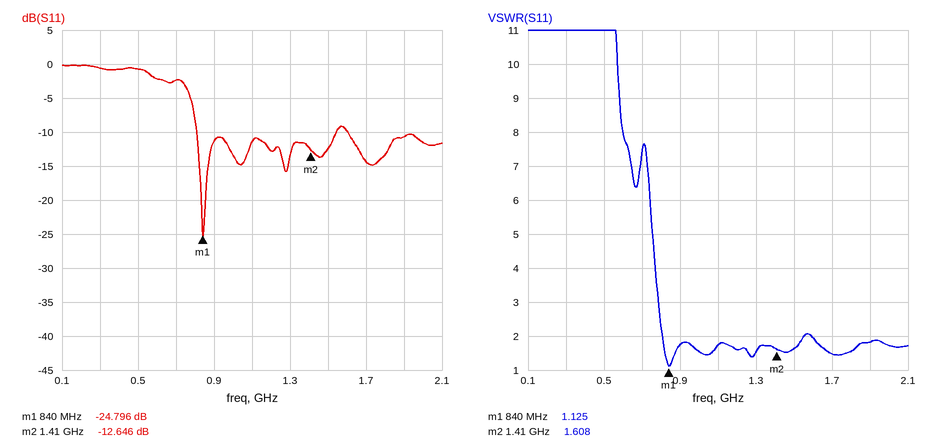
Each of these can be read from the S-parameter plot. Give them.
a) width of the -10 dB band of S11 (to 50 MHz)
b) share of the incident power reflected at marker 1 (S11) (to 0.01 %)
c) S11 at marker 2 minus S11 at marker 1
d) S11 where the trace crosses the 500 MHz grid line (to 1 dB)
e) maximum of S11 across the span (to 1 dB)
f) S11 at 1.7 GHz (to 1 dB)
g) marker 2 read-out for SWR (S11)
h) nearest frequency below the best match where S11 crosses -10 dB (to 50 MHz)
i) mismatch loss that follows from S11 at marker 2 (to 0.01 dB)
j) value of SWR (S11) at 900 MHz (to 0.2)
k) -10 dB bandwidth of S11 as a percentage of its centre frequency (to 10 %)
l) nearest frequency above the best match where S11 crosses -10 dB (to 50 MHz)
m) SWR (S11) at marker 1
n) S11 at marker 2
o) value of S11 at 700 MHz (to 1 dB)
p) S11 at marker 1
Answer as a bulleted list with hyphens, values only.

- 750 MHz
- 0.33 %
- 12.150 dB
- -1 dB
- 0 dB
- -14 dB
- 1.608
- 800 MHz
- 0.24 dB
- 1.8
- 60 %
- 1.55 GHz
- 1.125
- -12.646 dB
- -2 dB
- -24.796 dB
